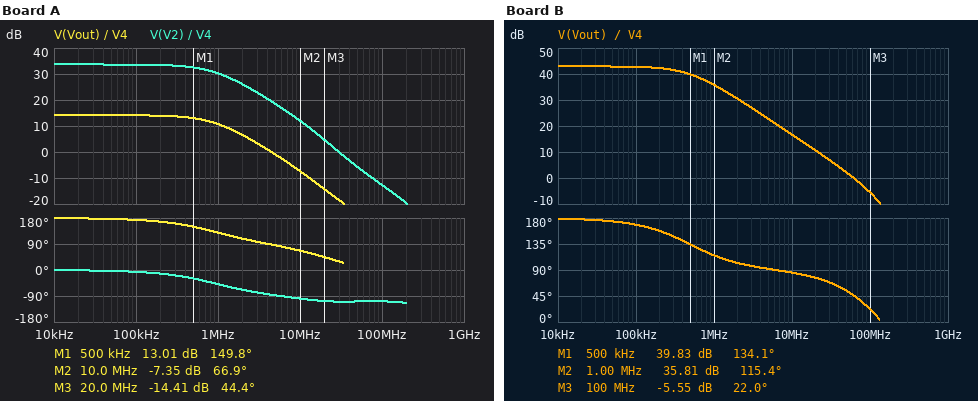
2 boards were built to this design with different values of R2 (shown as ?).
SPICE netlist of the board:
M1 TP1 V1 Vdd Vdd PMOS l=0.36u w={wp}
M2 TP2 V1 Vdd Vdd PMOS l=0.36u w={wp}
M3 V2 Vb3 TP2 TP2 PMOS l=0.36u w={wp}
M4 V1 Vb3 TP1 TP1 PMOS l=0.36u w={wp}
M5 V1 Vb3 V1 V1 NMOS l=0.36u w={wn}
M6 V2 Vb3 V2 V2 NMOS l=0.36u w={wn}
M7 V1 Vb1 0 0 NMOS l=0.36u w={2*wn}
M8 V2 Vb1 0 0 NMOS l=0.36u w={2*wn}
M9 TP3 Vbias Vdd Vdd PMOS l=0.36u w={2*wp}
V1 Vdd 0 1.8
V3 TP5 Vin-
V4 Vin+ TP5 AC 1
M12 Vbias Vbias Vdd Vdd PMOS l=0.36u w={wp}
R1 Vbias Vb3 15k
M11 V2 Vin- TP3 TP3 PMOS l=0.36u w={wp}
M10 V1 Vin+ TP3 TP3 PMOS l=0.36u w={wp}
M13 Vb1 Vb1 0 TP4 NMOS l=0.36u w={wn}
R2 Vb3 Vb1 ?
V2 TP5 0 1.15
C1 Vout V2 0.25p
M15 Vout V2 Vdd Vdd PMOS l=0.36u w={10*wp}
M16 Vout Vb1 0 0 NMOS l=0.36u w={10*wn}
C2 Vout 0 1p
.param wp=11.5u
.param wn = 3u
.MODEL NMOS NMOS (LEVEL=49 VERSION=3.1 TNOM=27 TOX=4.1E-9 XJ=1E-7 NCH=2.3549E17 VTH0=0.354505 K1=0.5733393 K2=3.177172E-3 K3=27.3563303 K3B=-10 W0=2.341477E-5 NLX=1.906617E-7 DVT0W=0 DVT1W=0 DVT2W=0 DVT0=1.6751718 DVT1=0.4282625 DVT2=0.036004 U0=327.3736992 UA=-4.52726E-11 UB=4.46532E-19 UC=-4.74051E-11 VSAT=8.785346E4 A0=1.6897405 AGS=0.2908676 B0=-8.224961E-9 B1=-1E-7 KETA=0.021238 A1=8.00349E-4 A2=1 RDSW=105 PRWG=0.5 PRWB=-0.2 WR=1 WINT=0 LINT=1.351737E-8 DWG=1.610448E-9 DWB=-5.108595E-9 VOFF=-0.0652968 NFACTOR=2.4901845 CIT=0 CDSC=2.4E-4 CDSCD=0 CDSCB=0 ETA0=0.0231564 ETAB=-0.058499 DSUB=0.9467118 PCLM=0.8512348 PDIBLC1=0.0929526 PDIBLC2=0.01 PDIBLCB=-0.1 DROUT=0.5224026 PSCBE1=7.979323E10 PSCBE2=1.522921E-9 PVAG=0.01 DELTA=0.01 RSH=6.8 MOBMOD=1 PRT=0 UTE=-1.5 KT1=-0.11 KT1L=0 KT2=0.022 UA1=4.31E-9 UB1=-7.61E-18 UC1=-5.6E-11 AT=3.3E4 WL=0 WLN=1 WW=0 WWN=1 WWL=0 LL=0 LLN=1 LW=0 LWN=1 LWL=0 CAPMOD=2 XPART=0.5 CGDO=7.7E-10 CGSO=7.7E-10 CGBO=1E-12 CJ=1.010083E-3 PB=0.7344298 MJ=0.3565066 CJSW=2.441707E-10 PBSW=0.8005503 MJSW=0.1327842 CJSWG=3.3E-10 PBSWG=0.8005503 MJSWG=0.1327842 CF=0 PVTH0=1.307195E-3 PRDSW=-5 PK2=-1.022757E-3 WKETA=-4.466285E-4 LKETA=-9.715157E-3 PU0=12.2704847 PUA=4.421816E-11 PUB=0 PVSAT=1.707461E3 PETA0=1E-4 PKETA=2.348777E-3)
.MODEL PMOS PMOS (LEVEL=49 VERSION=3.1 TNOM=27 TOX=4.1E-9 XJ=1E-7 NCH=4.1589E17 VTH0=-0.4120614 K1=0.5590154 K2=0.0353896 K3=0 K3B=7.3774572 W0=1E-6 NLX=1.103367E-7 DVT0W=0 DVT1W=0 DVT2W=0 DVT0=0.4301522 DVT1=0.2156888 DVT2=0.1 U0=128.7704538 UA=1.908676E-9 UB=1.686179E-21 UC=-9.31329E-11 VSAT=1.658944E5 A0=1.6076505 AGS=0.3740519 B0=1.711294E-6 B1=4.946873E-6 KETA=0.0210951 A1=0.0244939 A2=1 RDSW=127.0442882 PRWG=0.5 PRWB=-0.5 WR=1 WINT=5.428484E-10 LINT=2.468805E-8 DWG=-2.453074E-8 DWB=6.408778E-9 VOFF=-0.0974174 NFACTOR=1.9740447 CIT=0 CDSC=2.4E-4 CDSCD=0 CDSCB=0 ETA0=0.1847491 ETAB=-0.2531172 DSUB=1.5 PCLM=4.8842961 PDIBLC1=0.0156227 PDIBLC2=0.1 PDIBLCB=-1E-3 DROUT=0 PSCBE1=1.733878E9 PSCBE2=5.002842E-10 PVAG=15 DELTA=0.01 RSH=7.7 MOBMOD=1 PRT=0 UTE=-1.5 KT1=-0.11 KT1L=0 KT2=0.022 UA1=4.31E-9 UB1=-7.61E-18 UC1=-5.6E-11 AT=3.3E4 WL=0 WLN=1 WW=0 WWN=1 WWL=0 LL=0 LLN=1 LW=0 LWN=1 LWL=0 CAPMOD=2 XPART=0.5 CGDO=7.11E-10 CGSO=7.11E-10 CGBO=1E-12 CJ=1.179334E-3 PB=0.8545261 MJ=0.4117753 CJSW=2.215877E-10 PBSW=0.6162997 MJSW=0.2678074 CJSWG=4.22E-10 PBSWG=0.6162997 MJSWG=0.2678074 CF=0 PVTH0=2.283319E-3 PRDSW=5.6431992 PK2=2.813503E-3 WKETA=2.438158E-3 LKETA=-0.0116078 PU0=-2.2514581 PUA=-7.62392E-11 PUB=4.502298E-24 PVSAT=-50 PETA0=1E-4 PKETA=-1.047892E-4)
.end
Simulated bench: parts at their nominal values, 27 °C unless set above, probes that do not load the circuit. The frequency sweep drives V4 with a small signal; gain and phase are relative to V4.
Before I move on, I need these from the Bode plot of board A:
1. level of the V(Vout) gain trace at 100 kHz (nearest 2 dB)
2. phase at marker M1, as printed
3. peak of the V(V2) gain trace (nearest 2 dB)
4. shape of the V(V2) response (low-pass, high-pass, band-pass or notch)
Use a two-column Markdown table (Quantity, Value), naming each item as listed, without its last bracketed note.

| Quantity | Value |
|---|---|
| level of the V(Vout) gain trace at 100 kHz | 14 dB |
| phase at marker M1, as printed | 149.8 deg |
| peak of the V(V2) gain trace | 34 dB |
| shape of the V(V2) response | low-pass |
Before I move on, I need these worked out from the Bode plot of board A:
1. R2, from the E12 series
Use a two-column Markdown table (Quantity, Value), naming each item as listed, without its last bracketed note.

| Quantity | Value |
|---|---|
| R2, from the E12 series | 22 kΩ |
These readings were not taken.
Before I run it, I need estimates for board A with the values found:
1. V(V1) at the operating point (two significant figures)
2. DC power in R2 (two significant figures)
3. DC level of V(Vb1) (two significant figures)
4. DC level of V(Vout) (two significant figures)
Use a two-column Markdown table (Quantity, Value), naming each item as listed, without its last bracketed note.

| Quantity | Value |
|---|---|
| V(V1) at the operating point | 1.4 V |
| DC power in R2 | 6.9 µW |
| DC level of V(Vb1) | 550 mV |
| DC level of V(Vout) | 4.5 mV |
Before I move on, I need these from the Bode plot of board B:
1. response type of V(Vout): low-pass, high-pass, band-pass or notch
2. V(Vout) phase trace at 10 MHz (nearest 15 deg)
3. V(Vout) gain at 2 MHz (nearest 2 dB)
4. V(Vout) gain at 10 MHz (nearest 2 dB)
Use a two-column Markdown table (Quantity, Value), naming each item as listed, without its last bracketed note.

| Quantity | Value |
|---|---|
| response type of V(Vout): low-pass, high-pass, band-pass or notch | low-pass |
| V(Vout) phase trace at 10 MHz | 90 deg |
| V(Vout) gain at 2 MHz | 30 dB |
| V(Vout) gain at 10 MHz | 16 dB |
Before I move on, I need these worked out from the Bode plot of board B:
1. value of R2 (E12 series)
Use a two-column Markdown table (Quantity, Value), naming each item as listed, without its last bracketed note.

| Quantity | Value |
|---|---|
| value of R2 | 4.7 kΩ |
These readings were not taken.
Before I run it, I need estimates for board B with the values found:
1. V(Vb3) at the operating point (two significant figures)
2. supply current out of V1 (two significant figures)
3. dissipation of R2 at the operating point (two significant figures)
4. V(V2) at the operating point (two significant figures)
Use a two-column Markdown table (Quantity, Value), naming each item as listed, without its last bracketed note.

| Quantity | Value |
|---|---|
| V(Vb3) at the operating point | 730 mV |
| supply current out of V1 | 170 µA |
| dissipation of R2 at the operating point | 4.1 µW |
| V(V2) at the operating point | 1.3 V |
